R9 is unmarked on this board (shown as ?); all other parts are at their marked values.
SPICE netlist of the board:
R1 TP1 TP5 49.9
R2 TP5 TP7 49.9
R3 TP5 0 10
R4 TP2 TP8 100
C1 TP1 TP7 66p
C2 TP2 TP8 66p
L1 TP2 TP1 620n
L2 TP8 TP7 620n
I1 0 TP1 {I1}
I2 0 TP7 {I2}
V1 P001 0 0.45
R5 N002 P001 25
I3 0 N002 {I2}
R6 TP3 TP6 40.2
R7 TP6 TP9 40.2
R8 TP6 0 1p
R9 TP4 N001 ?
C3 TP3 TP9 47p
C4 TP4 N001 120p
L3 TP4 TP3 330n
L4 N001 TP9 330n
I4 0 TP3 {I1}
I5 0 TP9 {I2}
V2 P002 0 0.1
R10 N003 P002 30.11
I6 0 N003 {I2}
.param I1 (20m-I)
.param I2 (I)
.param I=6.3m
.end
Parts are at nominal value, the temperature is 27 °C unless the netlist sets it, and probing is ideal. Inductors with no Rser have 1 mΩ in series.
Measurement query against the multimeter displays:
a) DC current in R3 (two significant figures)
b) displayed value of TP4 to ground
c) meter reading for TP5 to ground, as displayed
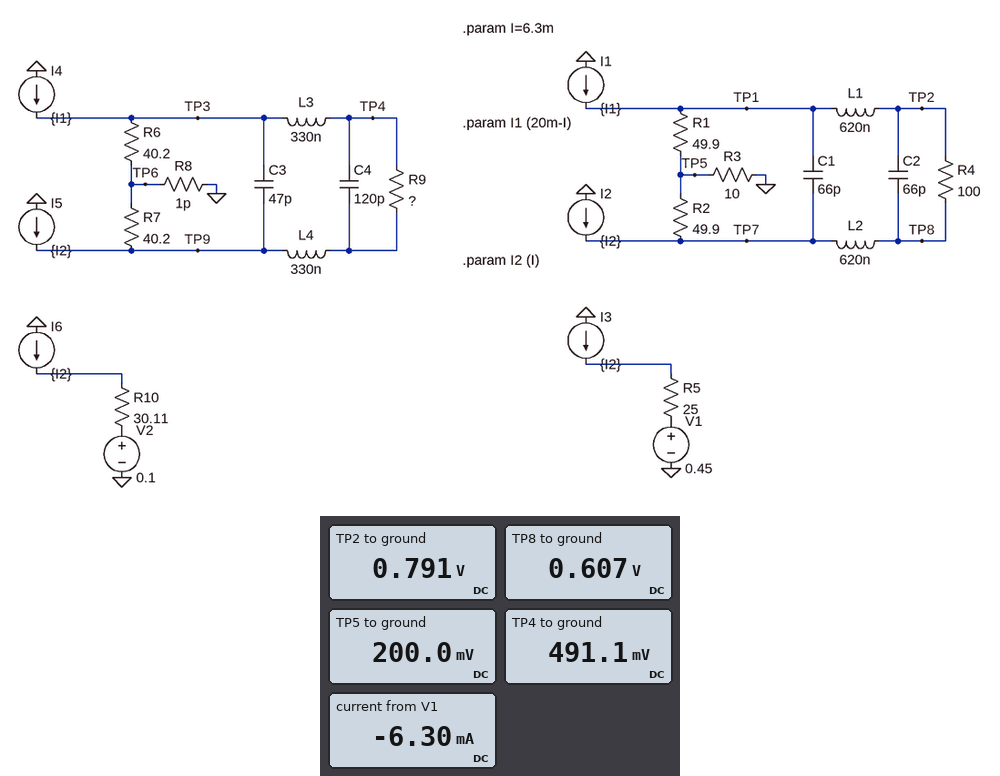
20 mA
491.1 mV
200.0 mV
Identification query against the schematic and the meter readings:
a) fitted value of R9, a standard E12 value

120 Ω
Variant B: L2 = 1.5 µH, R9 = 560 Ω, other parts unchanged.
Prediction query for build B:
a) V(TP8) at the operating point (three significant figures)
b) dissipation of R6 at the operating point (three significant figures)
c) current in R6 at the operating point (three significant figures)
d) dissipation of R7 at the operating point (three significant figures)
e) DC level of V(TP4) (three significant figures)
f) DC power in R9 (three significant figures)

607 mV
7.04 mW
13.2 mA
1.84 mW
532 mV
121 µW
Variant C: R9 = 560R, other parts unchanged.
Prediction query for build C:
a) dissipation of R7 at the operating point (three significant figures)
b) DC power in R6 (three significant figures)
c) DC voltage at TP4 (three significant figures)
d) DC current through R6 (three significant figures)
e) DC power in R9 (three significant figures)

1.84 mW
7.04 mW
532 mV
13.2 mA
121 µW
